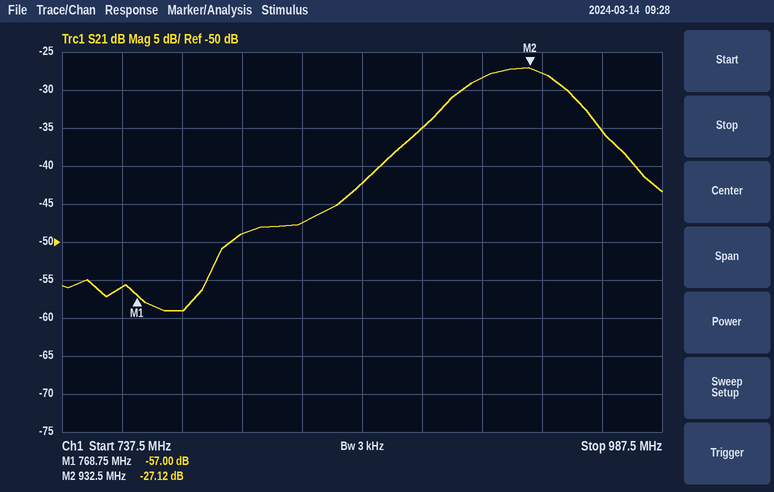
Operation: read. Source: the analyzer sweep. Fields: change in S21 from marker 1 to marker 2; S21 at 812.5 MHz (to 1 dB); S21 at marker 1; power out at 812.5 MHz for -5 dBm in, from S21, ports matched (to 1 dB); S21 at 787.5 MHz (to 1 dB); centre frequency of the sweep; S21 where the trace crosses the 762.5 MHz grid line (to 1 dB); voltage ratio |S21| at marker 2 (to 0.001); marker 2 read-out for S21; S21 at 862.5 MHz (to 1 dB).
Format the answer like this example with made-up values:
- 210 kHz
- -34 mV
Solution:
- 29.88 dB
- -49 dB
- -57.00 dB
- -54 dBm
- -59 dB
- 862.5 MHz
- -56 dB
- 0.044
- -27.12 dB
- -42 dB
